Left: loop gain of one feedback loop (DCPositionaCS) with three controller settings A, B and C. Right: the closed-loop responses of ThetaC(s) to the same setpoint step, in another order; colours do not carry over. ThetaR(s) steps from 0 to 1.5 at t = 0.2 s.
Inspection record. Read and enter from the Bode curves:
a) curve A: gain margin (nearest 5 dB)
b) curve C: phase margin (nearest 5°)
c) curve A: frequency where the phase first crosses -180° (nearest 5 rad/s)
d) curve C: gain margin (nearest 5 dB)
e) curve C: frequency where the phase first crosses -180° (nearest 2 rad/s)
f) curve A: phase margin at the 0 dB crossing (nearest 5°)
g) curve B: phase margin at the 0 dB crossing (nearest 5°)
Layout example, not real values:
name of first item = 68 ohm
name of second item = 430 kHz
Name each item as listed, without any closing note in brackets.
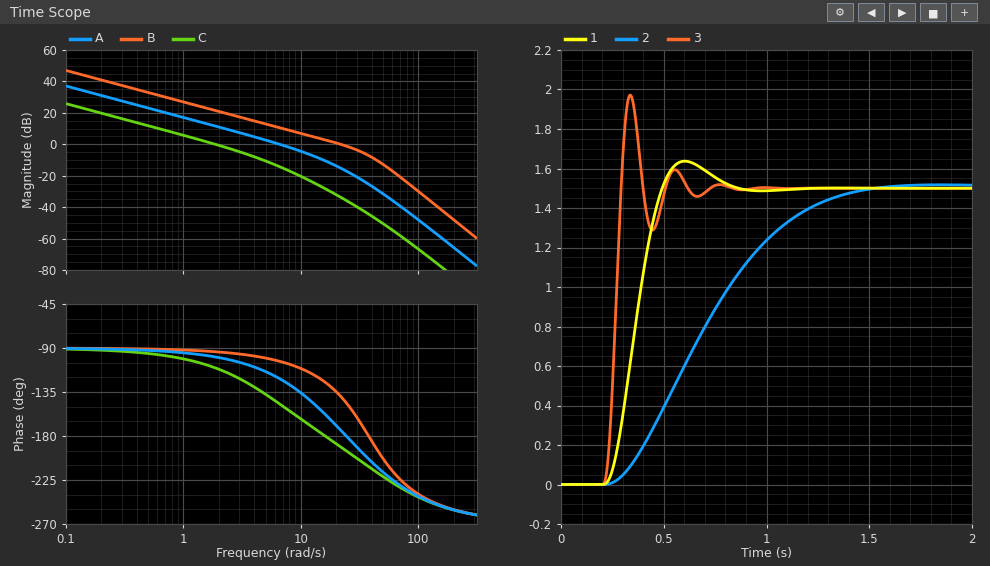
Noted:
curve A: gain margin = 15 dB
curve C: phase margin = 70°
curve A: frequency where the phase first crosses -180° = 25 rad/s
curve C: gain margin = 30 dB
curve C: frequency where the phase first crosses -180° = 16 rad/s
curve A: phase margin at the 0 dB crossing = 60°
curve B: phase margin at the 0 dB crossing = 40°
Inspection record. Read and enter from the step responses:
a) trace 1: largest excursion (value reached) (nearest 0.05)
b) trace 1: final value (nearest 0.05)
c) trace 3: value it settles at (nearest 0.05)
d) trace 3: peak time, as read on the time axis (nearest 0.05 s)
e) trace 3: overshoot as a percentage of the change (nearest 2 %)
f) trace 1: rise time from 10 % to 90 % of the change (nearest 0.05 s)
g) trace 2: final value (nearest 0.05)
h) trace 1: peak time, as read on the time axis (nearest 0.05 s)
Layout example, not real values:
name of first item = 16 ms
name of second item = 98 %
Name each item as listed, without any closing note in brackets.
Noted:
trace 1: largest excursion (value reached) = 1.65
trace 1: final value = 1.50
trace 3: value it settles at = 1.50
trace 3: peak time, as read on the time axis = 0.35 s
trace 3: overshoot as a percentage of the change = 32 %
trace 1: rise time from 10 % to 90 % of the change = 0.20 s
trace 2: final value = 1.50
trace 1: peak time, as read on the time axis = 0.60 s
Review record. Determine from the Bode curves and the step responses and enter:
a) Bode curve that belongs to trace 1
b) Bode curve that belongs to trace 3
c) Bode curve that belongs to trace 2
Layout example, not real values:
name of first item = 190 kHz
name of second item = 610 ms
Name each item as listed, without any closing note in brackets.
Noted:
Bode curve that belongs to trace 1 = A
Bode curve that belongs to trace 3 = B
Bode curve that belongs to trace 2 = C
